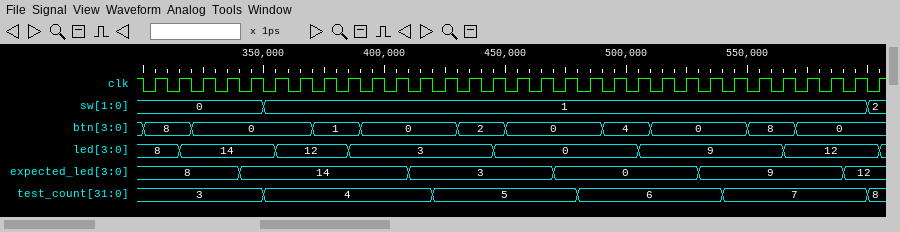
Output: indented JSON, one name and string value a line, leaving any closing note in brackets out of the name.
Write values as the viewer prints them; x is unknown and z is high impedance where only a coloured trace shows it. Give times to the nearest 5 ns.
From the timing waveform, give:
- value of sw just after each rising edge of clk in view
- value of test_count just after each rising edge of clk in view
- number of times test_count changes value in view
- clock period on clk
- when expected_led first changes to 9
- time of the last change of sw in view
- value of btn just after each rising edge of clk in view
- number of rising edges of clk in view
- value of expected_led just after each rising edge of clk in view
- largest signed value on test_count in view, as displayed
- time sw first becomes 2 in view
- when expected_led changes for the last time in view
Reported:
{
  "value of sw just after each rising edge of clk in view": "0, 0, 0, 0, 0, 1, 1, 1, 1, 1, 1, 1, 1, 1, 1, 1, 1, 1, 1, 1, 1, 1, 1, 1, 1, 1, 1, 1, 1, 1, 2",
  "value of test_count just after each rising edge of clk in view": "3, 3, 3, 3, 3, 4, 4, 4, 4, 4, 4, 4, 5, 5, 5, 5, 5, 5, 6, 6, 6, 6, 6, 6, 7, 7, 7, 7, 7, 7, 8",
  "number of times test_count changes value in view": "5",
  "clock period on clk": "10 ns",
  "when expected_led first changes to 9": "530 ns",
  "time of the last change of sw in view": "600 ns",
  "value of btn just after each rising edge of clk in view": "8, 8, 0, 0, 0, 0, 0, 1, 1, 0, 0, 0, 0, 2, 2, 0, 0, 0, 0, 4, 4, 0, 0, 0, 0, 8, 8, 0, 0, 0, 0",
  "number of rising edges of clk in view": "31",
  "value of expected_led just after each rising edge of clk in view": "8, 8, 8, 8, 14, 14, 14, 14, 14, 14, 14, 3, 3, 3, 3, 3, 3, 0, 0, 0, 0, 0, 0, 9, 9, 9, 9, 9, 9, 12, 12",
  "largest signed value on test_count in view, as displayed": "8",
  "time sw first becomes 2 in view": "600 ns",
  "when expected_led changes for the last time in view": "590 ns"
}
